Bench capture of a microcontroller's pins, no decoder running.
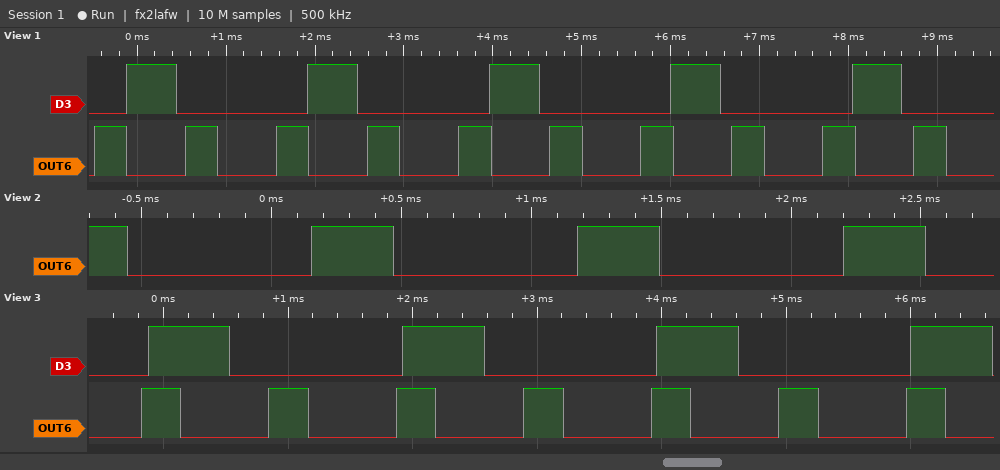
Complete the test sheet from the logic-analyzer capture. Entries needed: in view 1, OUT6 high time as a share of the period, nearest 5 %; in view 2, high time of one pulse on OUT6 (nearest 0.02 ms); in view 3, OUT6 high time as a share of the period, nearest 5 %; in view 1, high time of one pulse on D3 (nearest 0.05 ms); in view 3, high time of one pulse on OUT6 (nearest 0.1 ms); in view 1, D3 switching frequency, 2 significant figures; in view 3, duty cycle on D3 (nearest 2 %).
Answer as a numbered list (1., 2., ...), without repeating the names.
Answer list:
1. 35 %
2. 0.32 ms
3. 30 %
4. 0.55 ms
5. 0.3 ms
6. 490 Hz
7. 32 %
